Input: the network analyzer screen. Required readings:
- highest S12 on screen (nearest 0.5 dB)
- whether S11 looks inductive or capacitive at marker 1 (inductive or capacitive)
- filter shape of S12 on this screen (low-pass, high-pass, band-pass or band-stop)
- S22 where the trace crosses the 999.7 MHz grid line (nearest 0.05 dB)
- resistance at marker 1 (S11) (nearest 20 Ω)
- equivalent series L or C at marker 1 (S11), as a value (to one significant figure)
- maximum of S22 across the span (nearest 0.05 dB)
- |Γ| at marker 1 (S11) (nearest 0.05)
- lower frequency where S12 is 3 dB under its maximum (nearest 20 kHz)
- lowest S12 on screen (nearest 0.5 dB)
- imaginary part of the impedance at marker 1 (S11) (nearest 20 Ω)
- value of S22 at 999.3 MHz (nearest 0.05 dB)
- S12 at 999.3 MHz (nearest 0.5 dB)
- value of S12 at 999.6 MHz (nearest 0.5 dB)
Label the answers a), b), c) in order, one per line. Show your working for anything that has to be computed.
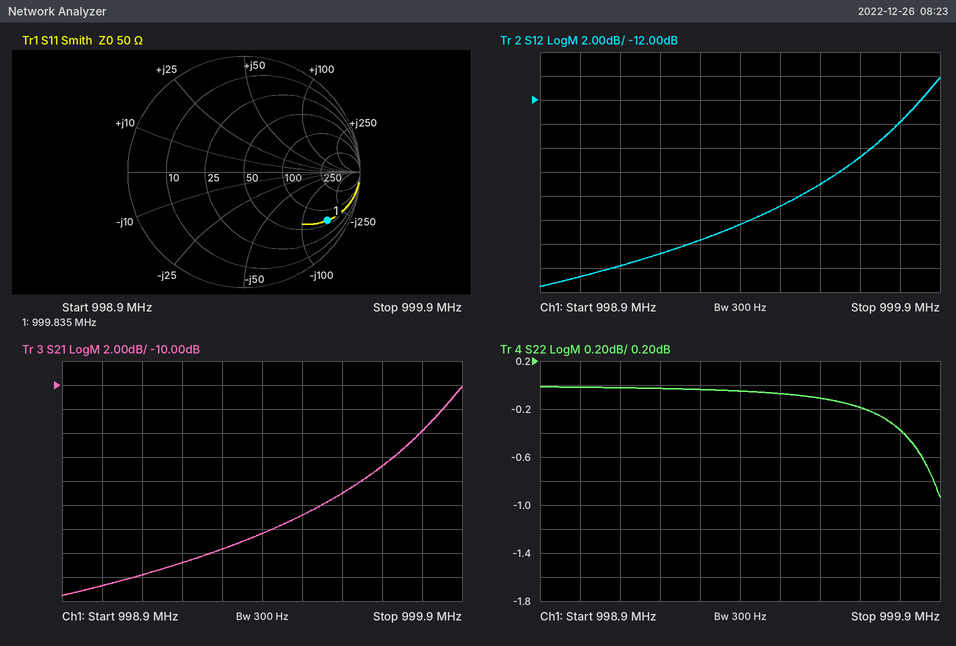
a) -10.0 dB
b) capacitive
c) high-pass
d) -0.20 dB
e) 60 Ω
f) C = 1/(2π × 999.835 MHz × 160 Ω) ≈ 1.0 pF
g) 0.00 dB
h) 0.85
i) 999.82 MHz
j) -27.5 dB
k) -160 Ω
l) -0.05 dB
m) -23.5 dB
n) -19.0 dB
